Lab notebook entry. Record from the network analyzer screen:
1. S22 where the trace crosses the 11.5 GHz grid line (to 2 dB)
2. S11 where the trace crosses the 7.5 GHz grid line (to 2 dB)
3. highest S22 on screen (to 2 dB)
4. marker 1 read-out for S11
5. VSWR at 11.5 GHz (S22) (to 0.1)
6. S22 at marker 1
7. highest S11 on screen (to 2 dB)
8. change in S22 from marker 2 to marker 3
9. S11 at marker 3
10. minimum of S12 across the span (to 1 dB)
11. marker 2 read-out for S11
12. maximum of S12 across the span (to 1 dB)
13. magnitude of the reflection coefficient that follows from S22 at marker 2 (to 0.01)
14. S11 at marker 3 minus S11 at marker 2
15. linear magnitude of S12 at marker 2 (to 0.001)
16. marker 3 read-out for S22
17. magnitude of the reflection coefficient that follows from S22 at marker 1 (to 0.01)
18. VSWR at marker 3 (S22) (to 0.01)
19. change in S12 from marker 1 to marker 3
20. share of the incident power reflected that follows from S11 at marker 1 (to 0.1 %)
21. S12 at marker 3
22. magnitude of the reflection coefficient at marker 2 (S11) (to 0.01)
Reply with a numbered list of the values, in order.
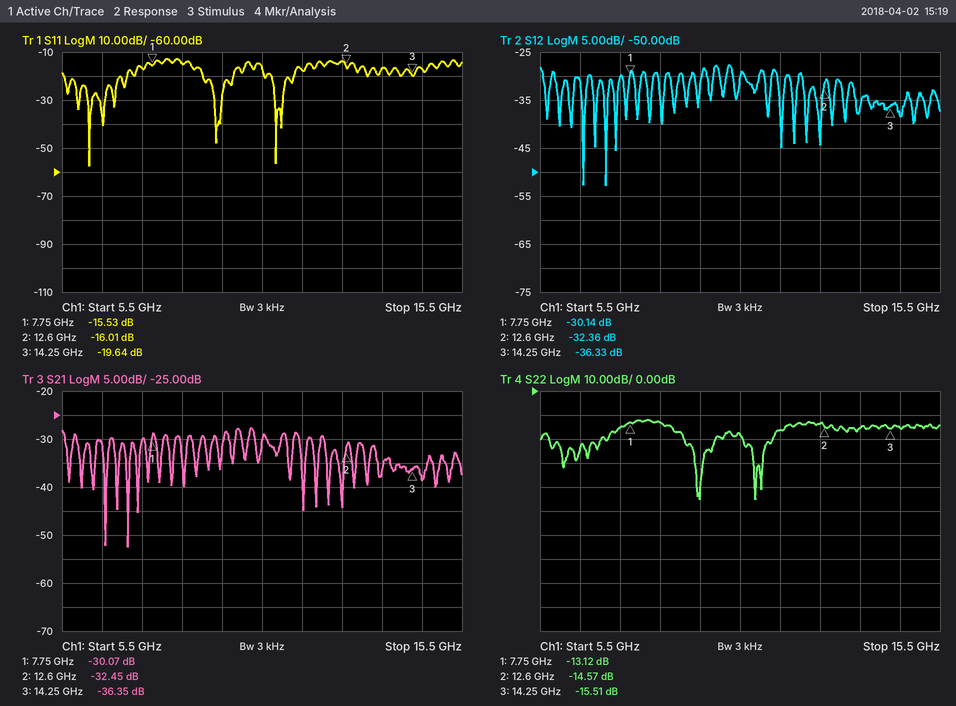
1. -16 dB
2. -16 dB
3. -12 dB
4. -15.53 dB
5. 1.4
6. -13.12 dB
7. -12 dB
8. -0.94 dB
9. -19.64 dB
10. -53 dB
11. -16.01 dB
12. -28 dB
13. 0.19
14. -3.63 dB
15. 0.024
16. -15.51 dB
17. 0.22
18. 1.40
19. -6.19 dB
20. 2.8 %
21. -36.33 dB
22. 0.16
